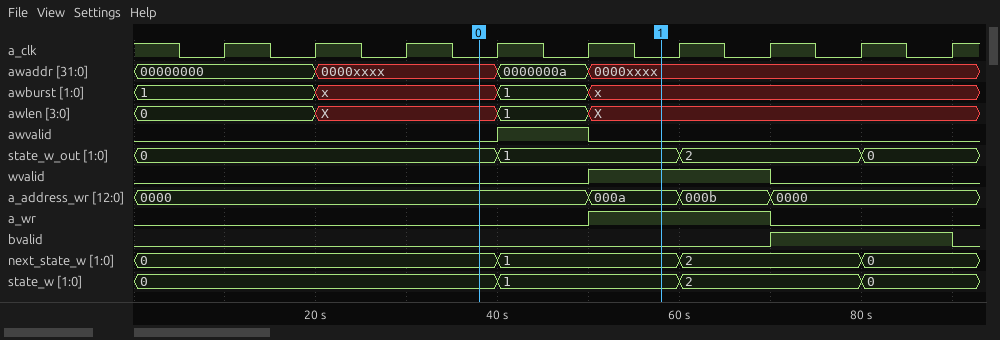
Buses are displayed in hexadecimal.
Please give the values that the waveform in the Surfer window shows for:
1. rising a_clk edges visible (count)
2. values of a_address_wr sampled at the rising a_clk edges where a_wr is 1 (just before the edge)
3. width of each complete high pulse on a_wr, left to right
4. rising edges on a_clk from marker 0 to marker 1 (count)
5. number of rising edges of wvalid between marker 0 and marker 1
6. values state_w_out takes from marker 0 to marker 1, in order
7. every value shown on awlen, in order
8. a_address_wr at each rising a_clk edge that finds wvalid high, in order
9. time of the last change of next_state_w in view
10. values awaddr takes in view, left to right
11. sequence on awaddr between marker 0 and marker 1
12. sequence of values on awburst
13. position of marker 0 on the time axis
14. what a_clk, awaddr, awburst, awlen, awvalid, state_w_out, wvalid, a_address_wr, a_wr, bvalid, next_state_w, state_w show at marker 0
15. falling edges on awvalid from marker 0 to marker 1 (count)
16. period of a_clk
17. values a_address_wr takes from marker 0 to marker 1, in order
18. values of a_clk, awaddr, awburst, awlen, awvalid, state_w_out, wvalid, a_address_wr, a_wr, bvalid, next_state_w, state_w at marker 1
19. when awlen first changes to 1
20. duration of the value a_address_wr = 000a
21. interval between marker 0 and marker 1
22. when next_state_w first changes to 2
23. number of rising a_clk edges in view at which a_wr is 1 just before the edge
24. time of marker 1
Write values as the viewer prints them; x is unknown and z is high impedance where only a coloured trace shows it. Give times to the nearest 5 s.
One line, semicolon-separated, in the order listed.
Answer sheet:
9; 000a, 000b; 20 s; 2; 1; 0, 1; 0, X, 1, X; 000a, 000b; 80 s; 00000000, 0000xxxx, 0000000a, 0000xxxx; 0000xxxx, 0000000a, 0000xxxx; 1, x, 1, x; 40 s; a_clk=0, awaddr=0000xxxx, awburst=x, awlen=X, awvalid=0, state_w_out=0, wvalid=0, a_address_wr=0000, a_wr=0, bvalid=0, next_state_w=0, state_w=0; 1; 10 s; 0000, 000a; a_clk=0, awaddr=0000xxxx, awburst=x, awlen=X, awvalid=0, state_w_out=1, wvalid=1, a_address_wr=000a, a_wr=1, bvalid=0, next_state_w=1, state_w=1; 40 s; 10 s; 20 s; 60 s; 2; 60 s
